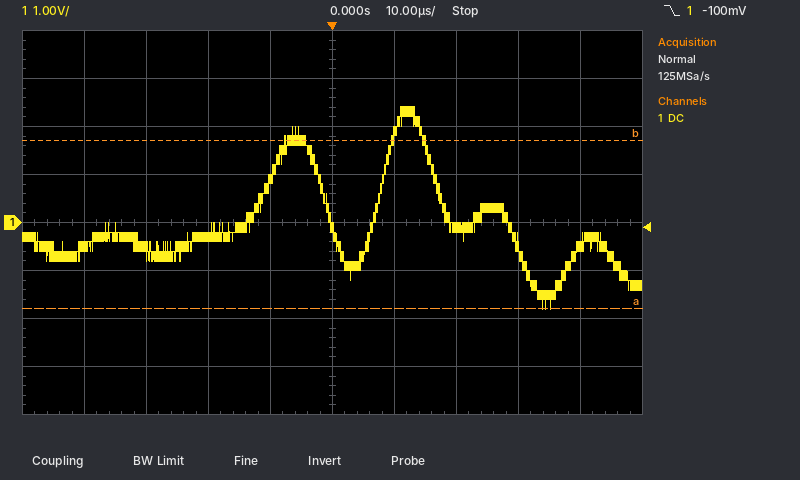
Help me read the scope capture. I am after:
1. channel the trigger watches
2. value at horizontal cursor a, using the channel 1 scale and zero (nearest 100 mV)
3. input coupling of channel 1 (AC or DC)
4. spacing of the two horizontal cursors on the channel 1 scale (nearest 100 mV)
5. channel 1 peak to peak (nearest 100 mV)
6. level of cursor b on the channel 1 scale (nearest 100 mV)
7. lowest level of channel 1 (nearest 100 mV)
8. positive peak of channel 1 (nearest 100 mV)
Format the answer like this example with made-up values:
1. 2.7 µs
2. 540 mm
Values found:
1. channel 1
2. -1.8 V
3. DC
4. 3.5 V
5. 4.2 V
6. 1.7 V
7. -1.8 V
8. 2.4 V
